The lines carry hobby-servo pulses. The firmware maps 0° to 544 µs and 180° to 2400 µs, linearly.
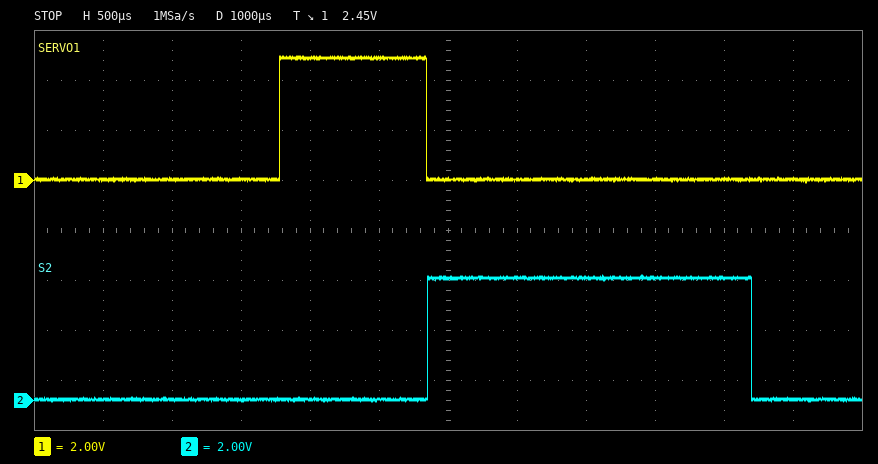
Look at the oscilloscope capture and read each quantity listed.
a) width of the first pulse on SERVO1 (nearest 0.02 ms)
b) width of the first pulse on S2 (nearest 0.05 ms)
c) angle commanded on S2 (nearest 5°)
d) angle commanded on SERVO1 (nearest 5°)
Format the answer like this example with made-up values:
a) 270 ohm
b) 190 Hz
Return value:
a) 1.06 ms
b) 2.35 ms
c) 175°
d) 50°
